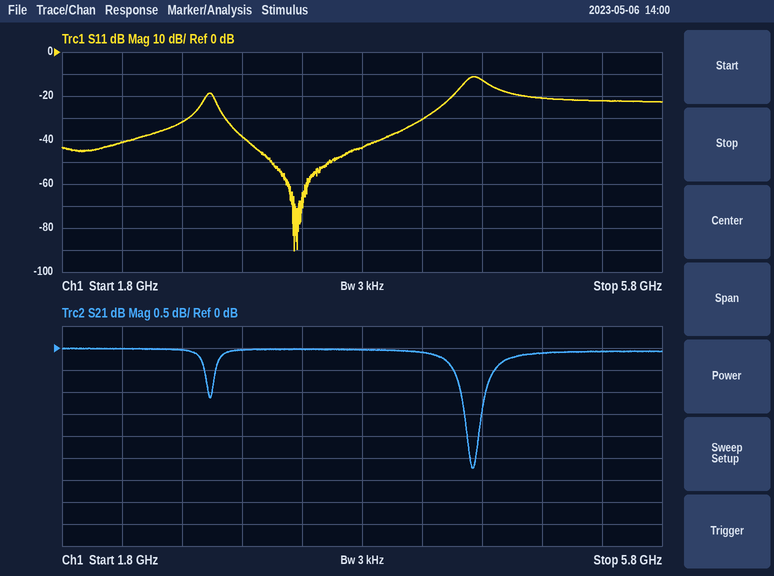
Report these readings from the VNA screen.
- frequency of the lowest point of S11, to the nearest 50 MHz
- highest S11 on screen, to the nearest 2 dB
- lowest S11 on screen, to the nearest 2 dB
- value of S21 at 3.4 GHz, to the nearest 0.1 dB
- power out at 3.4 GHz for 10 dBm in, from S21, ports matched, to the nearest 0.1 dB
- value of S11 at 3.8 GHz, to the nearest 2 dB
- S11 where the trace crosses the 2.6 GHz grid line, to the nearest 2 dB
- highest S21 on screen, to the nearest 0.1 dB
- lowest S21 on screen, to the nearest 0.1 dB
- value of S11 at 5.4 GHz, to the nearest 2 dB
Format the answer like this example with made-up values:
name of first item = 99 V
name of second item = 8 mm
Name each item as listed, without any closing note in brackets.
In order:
frequency of the lowest point of S11, to the nearest 50 MHz = 3.35 GHz
highest S11 on screen, to the nearest 2 dB = -12 dB
lowest S11 on screen, to the nearest 2 dB = -90 dB
value of S21 at 3.4 GHz, to the nearest 0.1 dB = 0.0 dB
power out at 3.4 GHz for 10 dBm in, from S21, ports matched, to the nearest 0.1 dB = 10.0 dBm
value of S11 at 3.8 GHz, to the nearest 2 dB = -44 dB
S11 where the trace crosses the 2.6 GHz grid line, to the nearest 2 dB = -32 dB
highest S21 on screen, to the nearest 0.1 dB = 0.0 dB
lowest S21 on screen, to the nearest 0.1 dB = -2.7 dB
value of S11 at 5.4 GHz, to the nearest 2 dB = -22 dB
